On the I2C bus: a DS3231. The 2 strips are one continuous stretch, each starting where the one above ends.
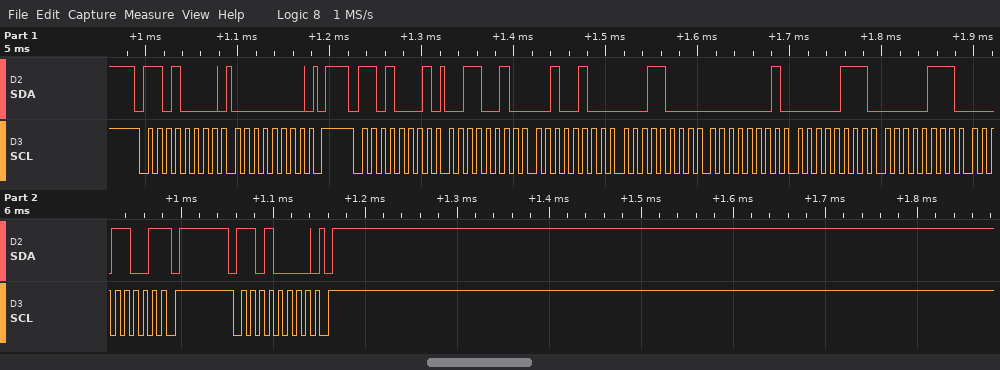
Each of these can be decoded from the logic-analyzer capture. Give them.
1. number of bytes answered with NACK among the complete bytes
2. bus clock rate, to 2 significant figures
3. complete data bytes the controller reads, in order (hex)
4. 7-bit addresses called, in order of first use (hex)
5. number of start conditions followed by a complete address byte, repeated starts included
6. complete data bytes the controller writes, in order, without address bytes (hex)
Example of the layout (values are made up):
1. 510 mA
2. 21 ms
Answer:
1. 1
2. 100 kHz
3. 32 24 18 01 07 07 19
4. 0x68
5. 3
6. 00
